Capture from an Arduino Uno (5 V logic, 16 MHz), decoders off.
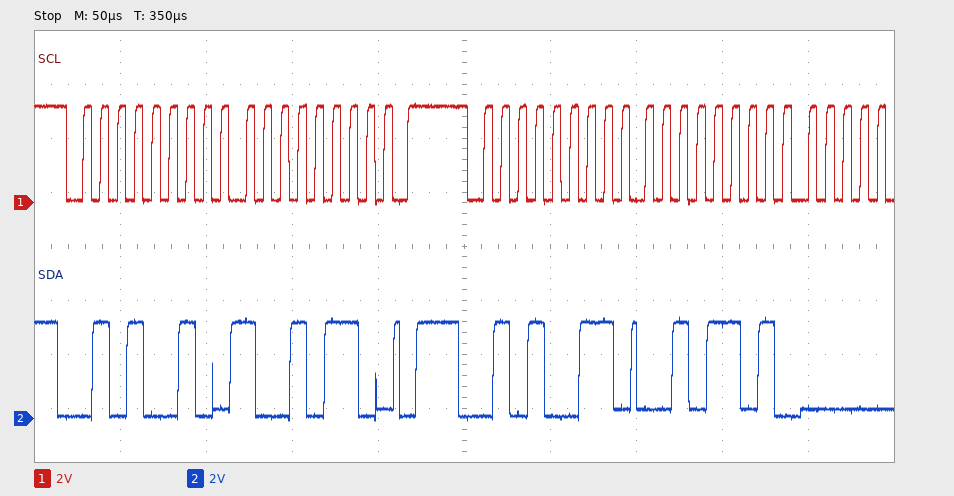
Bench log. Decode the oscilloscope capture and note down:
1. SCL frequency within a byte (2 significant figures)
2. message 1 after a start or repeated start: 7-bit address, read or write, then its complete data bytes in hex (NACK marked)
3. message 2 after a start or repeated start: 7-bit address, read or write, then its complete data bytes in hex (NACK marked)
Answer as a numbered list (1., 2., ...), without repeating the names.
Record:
1. 100 kHz
2. 0x29 write: 96
3. 0x29 read: 2D
